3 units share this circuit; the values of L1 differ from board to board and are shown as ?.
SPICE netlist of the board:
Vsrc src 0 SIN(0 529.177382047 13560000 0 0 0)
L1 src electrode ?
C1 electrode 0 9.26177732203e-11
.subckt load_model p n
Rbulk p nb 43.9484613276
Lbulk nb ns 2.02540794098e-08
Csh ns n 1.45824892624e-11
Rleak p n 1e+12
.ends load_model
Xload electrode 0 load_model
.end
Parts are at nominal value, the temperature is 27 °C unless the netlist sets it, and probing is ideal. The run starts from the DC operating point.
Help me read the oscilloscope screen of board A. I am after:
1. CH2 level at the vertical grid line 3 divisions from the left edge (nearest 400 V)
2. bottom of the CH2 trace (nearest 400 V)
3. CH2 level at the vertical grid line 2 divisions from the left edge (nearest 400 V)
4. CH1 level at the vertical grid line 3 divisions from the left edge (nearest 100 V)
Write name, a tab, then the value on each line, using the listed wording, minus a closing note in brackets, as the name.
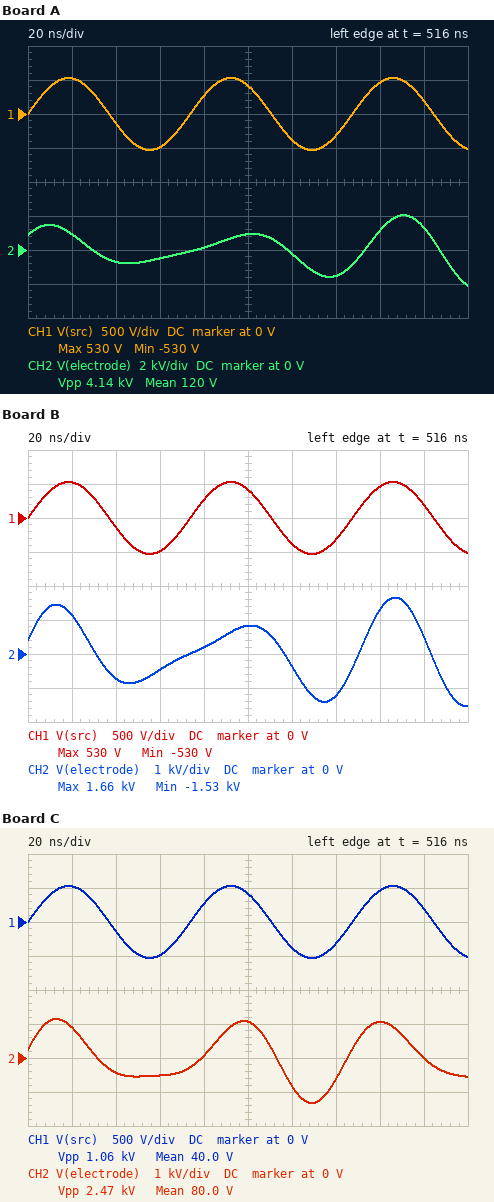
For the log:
CH2 level at the vertical grid line 3 divisions from the left edge	-400 V
bottom of the CH2 trace	-2.0 kV
CH2 level at the vertical grid line 2 divisions from the left edge	-800 V
CH1 level at the vertical grid line 3 divisions from the left edge	-500 V
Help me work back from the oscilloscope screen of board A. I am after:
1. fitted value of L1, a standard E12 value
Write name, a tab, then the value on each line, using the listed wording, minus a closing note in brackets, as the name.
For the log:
fitted value of L1, a standard E12 value	820 nH
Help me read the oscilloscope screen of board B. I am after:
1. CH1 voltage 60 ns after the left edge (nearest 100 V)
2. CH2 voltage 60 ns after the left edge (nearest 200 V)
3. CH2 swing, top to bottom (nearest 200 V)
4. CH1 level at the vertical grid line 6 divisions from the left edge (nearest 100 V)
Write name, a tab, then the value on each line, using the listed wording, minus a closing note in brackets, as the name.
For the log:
CH1 voltage 60 ns after the left edge	-500 V
CH2 voltage 60 ns after the left edge	-400 V
CH2 swing, top to bottom	3.2 kV
CH1 level at the vertical grid line 6 divisions from the left edge	-400 V
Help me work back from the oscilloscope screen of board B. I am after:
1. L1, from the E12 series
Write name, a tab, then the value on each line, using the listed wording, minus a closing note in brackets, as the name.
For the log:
L1, from the E12 series	680 nH
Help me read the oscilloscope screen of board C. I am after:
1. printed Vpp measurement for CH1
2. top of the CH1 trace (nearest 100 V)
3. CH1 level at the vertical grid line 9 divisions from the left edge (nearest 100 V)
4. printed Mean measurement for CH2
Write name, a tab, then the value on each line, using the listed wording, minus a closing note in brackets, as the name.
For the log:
printed Vpp measurement for CH1	1.06 kV
top of the CH1 trace	500 V
CH1 level at the vertical grid line 9 divisions from the left edge	200 V
printed Mean measurement for CH2	80.0 V
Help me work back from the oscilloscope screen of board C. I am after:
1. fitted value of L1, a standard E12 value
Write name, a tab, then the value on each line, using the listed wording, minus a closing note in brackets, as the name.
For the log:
fitted value of L1, a standard E12 value	560 nH
